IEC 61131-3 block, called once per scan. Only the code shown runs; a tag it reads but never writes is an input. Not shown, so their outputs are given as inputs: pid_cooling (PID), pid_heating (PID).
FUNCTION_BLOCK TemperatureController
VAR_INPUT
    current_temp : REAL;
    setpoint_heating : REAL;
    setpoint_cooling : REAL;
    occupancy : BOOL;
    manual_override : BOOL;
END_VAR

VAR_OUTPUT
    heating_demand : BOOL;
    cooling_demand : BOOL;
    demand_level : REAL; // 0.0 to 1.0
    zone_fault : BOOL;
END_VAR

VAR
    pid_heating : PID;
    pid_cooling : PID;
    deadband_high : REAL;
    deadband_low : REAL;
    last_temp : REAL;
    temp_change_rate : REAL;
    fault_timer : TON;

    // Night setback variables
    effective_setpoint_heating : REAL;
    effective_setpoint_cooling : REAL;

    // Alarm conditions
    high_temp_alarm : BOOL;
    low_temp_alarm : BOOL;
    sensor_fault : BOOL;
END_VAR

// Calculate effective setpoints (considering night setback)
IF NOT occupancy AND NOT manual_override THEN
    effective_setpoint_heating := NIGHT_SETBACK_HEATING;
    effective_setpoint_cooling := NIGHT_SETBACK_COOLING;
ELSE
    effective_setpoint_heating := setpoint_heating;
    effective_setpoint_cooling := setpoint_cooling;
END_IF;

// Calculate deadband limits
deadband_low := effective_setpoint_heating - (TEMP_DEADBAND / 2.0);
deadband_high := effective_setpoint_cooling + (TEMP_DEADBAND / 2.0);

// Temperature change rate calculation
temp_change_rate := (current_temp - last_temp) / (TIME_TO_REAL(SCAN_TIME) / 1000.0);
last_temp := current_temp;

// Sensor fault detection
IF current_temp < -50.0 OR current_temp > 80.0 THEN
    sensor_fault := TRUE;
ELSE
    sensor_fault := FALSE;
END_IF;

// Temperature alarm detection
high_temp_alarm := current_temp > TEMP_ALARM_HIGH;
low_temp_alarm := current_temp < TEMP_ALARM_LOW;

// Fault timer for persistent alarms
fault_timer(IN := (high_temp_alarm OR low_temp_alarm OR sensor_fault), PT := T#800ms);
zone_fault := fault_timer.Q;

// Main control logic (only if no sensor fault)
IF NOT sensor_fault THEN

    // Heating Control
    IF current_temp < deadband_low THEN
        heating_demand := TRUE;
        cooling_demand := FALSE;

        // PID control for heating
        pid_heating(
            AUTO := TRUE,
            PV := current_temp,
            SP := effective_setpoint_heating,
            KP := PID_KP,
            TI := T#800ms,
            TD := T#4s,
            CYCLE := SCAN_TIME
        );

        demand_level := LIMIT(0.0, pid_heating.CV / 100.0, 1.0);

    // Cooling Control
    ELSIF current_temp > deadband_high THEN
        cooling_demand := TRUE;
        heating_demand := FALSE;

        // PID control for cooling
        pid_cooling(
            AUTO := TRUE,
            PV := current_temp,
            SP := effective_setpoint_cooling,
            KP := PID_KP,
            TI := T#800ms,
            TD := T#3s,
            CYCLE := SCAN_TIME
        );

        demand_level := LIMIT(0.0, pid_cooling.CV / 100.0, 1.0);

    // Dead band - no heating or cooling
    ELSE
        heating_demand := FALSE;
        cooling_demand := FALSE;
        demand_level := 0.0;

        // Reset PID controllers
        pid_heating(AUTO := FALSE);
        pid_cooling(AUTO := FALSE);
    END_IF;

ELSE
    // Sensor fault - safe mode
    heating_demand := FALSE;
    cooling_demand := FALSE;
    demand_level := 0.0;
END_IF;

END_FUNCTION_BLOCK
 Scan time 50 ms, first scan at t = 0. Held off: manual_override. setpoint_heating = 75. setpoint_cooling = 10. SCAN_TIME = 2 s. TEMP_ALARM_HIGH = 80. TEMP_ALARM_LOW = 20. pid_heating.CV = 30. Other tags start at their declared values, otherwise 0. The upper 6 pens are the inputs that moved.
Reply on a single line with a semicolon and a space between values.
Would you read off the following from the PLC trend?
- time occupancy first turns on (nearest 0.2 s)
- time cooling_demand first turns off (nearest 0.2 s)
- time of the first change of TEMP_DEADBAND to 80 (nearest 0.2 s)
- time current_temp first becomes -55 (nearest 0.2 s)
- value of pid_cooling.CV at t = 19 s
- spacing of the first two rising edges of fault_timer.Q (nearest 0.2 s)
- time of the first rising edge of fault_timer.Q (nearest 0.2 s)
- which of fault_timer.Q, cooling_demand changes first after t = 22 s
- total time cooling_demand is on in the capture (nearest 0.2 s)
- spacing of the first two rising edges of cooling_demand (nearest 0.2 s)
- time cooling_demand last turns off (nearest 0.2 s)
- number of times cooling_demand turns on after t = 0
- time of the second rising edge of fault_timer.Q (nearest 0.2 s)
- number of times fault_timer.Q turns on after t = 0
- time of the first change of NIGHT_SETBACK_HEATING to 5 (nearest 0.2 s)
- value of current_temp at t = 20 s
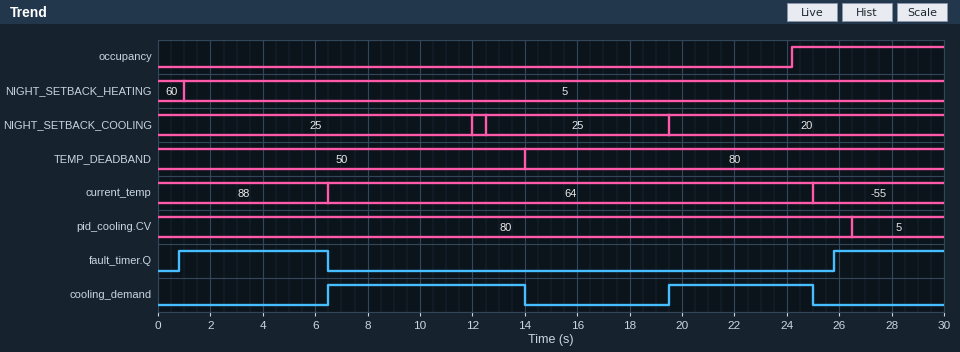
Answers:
24.2 s; 14.0 s; 14.0 s; 25.0 s; 80; 25.0 s; 0.8 s; cooling_demand; 13.0 s; 13.0 s; 25.0 s; 2; 25.8 s; 2; 1.0 s; 64
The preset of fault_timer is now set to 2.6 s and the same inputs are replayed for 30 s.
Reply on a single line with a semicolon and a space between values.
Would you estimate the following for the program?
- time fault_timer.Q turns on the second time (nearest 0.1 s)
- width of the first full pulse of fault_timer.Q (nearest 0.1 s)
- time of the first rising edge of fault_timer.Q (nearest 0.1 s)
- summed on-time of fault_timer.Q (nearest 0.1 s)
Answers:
27.6 s; 3.9 s; 2.6 s; 6.3 s
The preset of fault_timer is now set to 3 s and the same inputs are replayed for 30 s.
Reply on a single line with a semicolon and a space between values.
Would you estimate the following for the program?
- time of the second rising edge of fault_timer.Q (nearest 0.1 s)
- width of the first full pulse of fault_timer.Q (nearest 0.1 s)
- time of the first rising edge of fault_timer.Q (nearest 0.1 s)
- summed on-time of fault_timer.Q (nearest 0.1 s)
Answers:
28.0 s; 3.5 s; 3.0 s; 5.5 s
